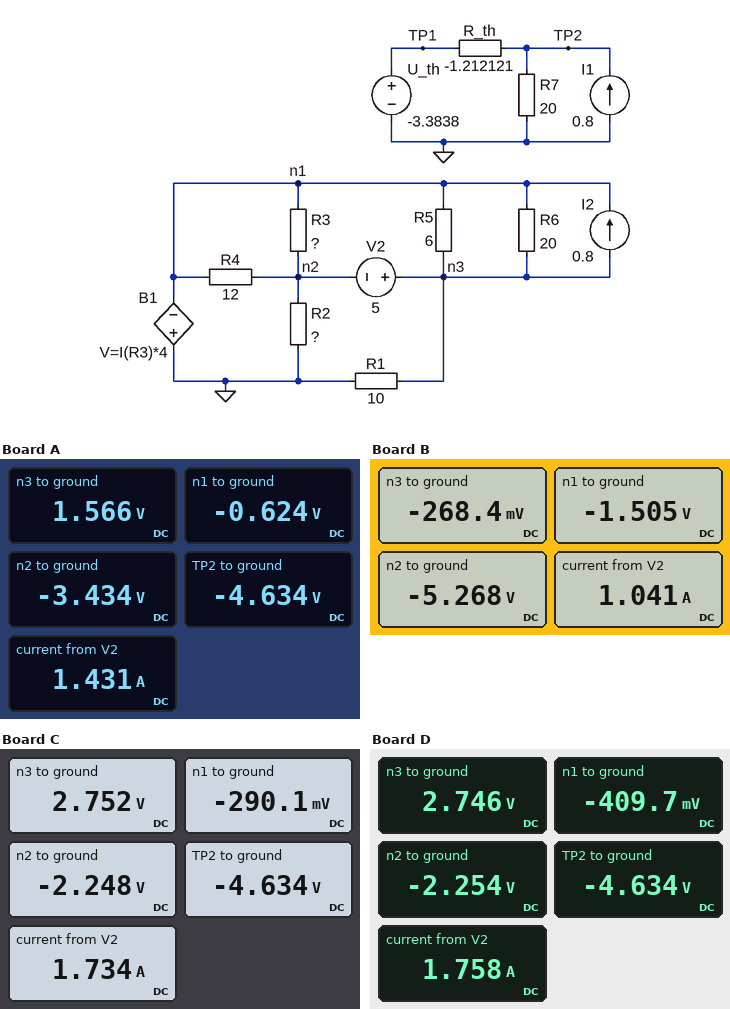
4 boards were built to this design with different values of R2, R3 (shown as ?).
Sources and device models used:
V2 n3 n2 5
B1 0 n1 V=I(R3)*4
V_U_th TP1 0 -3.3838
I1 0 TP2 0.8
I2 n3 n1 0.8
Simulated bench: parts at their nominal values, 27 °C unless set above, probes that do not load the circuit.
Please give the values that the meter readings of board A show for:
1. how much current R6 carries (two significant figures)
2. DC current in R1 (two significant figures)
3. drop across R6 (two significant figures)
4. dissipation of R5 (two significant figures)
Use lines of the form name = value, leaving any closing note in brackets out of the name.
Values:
how much current R6 carries = 110 mA
DC current in R1 = 160 mA
drop across R6 = 2.2 V
dissipation of R5 = 800 mW
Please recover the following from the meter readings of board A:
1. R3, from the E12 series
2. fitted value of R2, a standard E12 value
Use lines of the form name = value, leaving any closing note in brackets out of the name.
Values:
R3, from the E12 series = 18 Ω
fitted value of R2, a standard E12 value = 3.3 Ω
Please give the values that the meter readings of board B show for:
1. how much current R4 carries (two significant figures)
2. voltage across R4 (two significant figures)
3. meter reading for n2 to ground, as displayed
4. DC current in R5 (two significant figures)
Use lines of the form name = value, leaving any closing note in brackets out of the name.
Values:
how much current R4 carries = 310 mA
voltage across R4 = 3.8 V
meter reading for n2 to ground, as displayed = -5.268 V
DC current in R5 = 210 mA
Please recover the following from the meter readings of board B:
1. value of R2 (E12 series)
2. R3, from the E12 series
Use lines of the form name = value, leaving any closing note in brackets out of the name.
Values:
value of R2 = 15 Ω
R3, from the E12 series = 10 Ω
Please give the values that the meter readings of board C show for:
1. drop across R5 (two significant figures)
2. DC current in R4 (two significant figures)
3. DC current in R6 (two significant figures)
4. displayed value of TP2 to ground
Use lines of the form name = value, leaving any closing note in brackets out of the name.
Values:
drop across R5 = 3.0 V
DC current in R4 = 160 mA
DC current in R6 = 150 mA
displayed value of TP2 to ground = -4.634 V
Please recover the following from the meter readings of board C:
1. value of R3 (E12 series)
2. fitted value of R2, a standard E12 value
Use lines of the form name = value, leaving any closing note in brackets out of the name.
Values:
value of R3 = 27 Ω
fitted value of R2, a standard E12 value = 1.5 Ω
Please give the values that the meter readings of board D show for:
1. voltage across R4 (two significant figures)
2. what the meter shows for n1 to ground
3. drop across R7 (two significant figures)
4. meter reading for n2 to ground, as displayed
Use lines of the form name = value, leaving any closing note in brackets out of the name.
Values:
voltage across R4 = 1.8 V
what the meter shows for n1 to ground = -409.7 mV
drop across R7 = 4.6 V
meter reading for n2 to ground, as displayed = -2.254 V
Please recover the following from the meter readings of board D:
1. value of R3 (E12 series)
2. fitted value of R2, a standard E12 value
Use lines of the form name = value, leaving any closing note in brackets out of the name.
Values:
value of R3 = 18 Ω
fitted value of R2, a standard E12 value = 1.5 Ω
